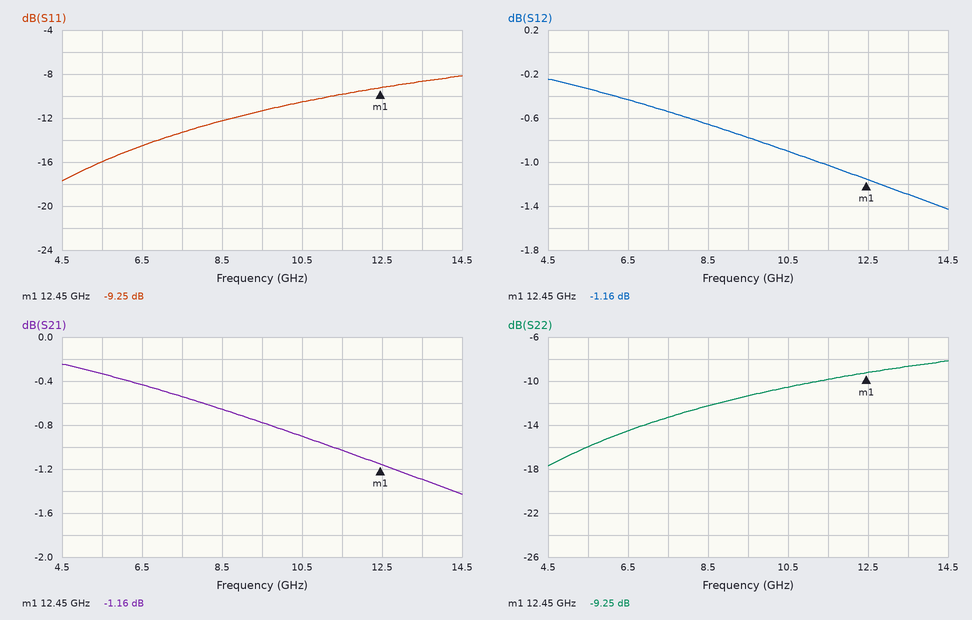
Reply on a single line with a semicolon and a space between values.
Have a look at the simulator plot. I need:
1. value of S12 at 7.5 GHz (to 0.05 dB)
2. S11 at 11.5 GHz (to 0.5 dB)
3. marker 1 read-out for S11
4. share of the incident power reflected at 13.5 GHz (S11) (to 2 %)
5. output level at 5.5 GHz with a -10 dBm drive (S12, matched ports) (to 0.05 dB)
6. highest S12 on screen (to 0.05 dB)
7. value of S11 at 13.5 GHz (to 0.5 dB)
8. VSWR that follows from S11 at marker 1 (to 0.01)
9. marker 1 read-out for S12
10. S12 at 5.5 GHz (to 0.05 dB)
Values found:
-0.55 dB; -10.0 dB; -9.25 dB; 14 %; -10.35 dBm; -0.25 dB; -8.5 dB; 2.05; -1.16 dB; -0.35 dB
